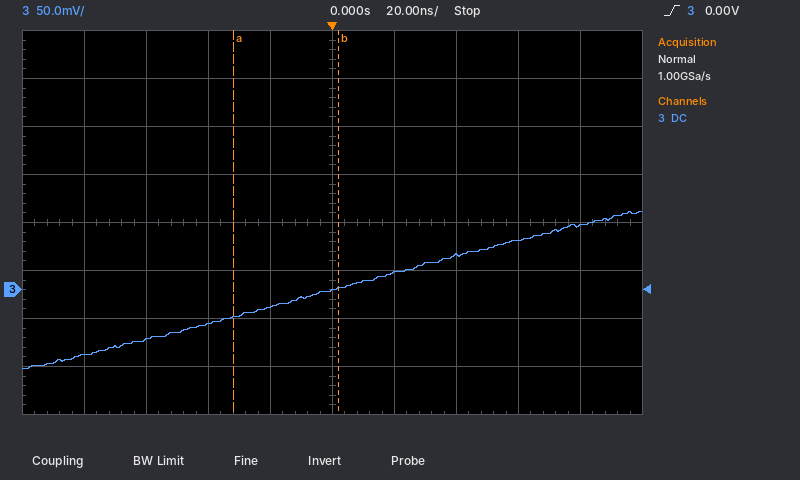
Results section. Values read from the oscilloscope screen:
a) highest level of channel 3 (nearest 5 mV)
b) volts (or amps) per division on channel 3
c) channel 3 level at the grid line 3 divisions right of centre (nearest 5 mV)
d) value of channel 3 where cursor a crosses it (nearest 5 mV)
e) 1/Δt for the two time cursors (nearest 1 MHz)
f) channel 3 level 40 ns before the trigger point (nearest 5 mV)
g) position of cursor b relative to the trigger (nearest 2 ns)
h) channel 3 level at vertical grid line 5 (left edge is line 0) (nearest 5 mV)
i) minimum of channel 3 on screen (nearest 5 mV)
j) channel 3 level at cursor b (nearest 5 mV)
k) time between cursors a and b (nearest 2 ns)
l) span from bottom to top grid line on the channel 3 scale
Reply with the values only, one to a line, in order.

80 mV
50 mV
50 mV
-30 mV
29 MHz
-35 mV
+2 ns
0 mV
-80 mV
0 mV
34 ns
400 mV
